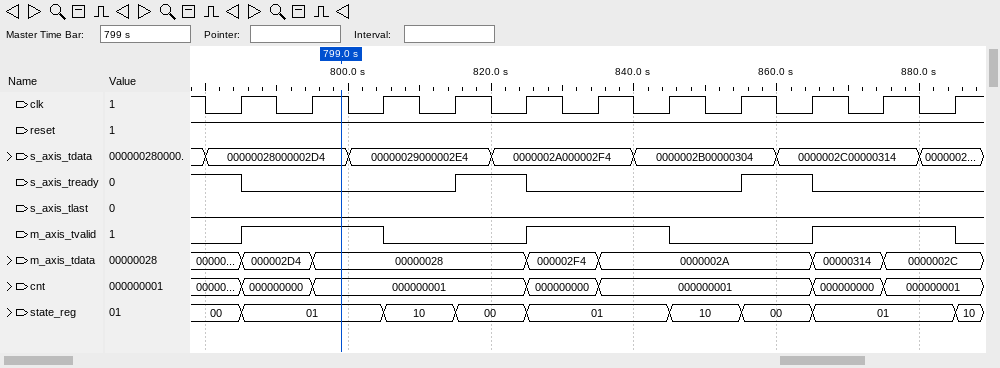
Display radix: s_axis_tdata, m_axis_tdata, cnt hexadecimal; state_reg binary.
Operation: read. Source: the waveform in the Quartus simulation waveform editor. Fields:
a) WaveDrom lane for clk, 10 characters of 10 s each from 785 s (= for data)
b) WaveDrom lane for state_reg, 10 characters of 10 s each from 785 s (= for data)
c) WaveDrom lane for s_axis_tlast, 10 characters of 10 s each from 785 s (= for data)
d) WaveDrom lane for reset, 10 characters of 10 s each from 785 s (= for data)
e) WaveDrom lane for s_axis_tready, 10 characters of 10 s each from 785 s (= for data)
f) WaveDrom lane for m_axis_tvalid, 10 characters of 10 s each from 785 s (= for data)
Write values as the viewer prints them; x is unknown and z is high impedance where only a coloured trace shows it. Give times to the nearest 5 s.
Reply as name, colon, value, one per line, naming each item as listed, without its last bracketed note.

WaveDrom lane for clk, 10 characters of 10 s each from 785 s: {name: 'clk', wave: 'p.........'}
WaveDrom lane for state_reg, 10 characters of 10 s each from 785 s: {name: 'state_reg', wave: '=.===.===.', data: '01 10 00 01 10 00 01'}
WaveDrom lane for s_axis_tlast, 10 characters of 10 s each from 785 s: {name: 's_axis_tlast', wave: '0.........'}
WaveDrom lane for reset, 10 characters of 10 s each from 785 s: {name: 'reset', wave: '1.........'}
WaveDrom lane for s_axis_tready, 10 characters of 10 s each from 785 s: {name: 's_axis_tready', wave: '0..10..10.'}
WaveDrom lane for m_axis_tvalid, 10 characters of 10 s each from 785 s: {name: 'm_axis_tvalid', wave: '1.0.1.0.1.'}
